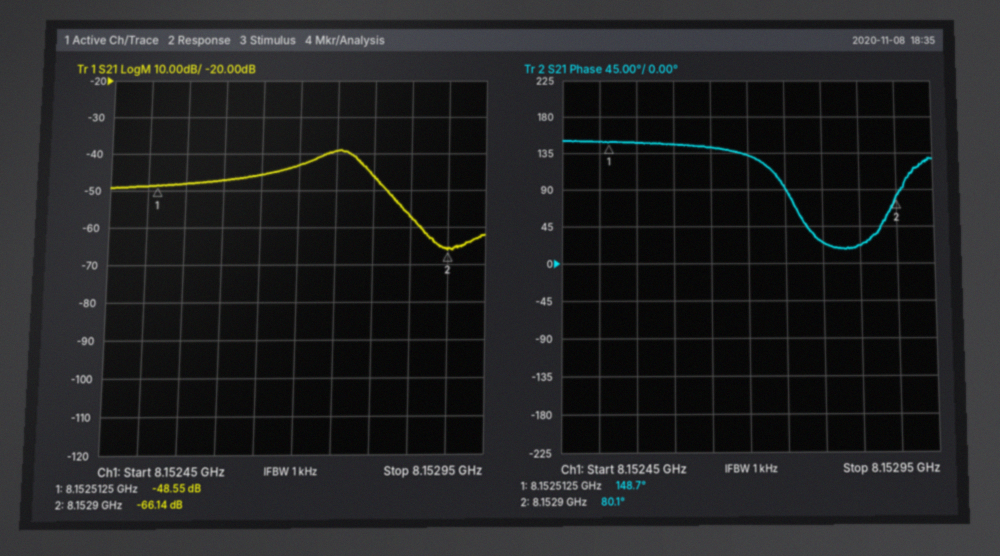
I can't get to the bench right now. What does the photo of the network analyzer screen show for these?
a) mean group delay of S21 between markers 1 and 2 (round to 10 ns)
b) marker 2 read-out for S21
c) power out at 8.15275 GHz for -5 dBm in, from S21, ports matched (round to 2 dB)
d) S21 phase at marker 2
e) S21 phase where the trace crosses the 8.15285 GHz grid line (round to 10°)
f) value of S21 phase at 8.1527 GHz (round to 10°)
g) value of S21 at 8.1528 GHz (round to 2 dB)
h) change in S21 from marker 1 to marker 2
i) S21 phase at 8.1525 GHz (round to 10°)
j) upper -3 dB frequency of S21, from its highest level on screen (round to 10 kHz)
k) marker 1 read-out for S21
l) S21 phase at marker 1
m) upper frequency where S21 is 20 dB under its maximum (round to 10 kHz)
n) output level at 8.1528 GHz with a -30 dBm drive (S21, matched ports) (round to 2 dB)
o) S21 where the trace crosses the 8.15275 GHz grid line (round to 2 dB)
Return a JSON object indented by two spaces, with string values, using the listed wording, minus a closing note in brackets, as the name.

{
  "mean group delay of S21 between markers 1 and 2": "490 ns",
  "marker 2 read-out for S21": "-66.14 dB",
  "power out at 8.15275 GHz for -5 dBm in, from S21, ports matched": "-44 dBm",
  "S21 phase at marker 2": "80.1°",
  "S21 phase where the trace crosses the 8.15285 GHz grid line": "20°",
  "value of S21 phase at 8.1527 GHz": "130°",
  "value of S21 at 8.1528 GHz": "-46 dB",
  "change in S21 from marker 1 to marker 2": "-17.59 dB",
  "S21 phase at 8.1525 GHz": "150°",
  "upper -3 dB frequency of S21, from its highest level on screen": "8.15278 GHz",
  "marker 1 read-out for S21": "-48.55 dB",
  "S21 phase at marker 1": "148.7°",
  "upper frequency where S21 is 20 dB under its maximum": "8.15286 GHz",
  "output level at 8.1528 GHz with a -30 dBm drive (S21, matched ports)": "-76 dBm",
  "S21 where the trace crosses the 8.15275 GHz grid line": "-40 dB"
}
